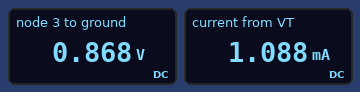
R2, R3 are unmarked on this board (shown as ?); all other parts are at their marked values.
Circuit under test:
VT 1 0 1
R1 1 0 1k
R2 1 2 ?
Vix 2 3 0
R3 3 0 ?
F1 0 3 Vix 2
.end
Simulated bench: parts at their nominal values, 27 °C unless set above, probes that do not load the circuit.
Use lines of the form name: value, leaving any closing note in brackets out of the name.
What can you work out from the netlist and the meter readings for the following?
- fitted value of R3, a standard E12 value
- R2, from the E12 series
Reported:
fitted value of R3, a standard E12 value: 3.3 kΩ
R2, from the E12 series: 1.5 kΩ
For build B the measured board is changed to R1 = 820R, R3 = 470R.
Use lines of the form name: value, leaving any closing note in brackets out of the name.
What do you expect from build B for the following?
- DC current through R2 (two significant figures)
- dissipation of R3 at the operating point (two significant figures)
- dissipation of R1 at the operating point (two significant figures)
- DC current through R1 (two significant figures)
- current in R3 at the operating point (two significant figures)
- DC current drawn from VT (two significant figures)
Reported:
DC current through R2: 340 µA
dissipation of R3 at the operating point: 500 µW
dissipation of R1 at the operating point: 1.2 mW
DC current through R1: 1.2 mA
current in R3 at the operating point: 1.0 mA
DC current drawn from VT: 1.6 mA
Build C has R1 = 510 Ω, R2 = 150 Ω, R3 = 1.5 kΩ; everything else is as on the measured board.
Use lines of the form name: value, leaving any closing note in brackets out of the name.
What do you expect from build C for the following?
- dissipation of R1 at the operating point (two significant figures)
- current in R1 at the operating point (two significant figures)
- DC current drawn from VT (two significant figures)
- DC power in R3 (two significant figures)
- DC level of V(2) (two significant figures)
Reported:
dissipation of R1 at the operating point: 2.0 mW
current in R1 at the operating point: 2.0 mA
DC current drawn from VT: 2.2 mA
DC power in R3: 620 µW
DC level of V(2): 970 mV
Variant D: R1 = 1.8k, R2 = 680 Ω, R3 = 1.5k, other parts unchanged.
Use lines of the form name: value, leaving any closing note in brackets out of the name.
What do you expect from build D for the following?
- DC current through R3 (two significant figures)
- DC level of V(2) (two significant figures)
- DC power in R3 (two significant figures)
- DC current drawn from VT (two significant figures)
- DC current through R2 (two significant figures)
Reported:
DC current through R3: 580 µA
DC level of V(2): 870 mV
DC power in R3: 500 µW
DC current drawn from VT: 750 µA
DC current through R2: 190 µA
